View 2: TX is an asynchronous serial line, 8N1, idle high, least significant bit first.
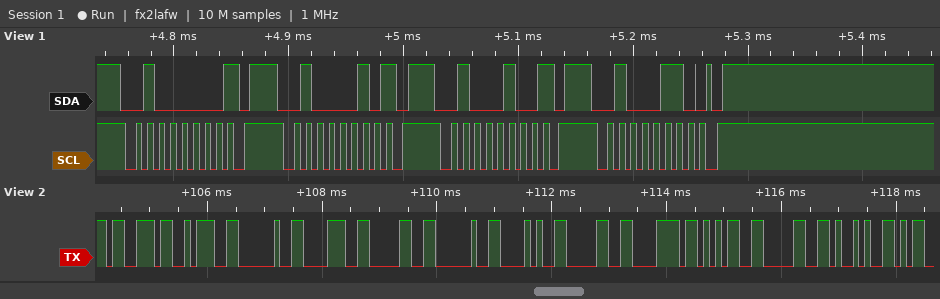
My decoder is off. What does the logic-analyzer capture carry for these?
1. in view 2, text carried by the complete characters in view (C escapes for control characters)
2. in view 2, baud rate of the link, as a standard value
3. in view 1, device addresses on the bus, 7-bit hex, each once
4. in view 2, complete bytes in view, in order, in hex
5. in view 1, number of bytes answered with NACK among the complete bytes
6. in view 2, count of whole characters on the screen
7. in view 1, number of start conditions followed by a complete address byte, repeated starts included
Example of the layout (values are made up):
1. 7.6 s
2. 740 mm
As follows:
1. "s: 80 (0x50)"
2. 9600 baud
3. 0x20 0x21 0x22 0x23
4. 73 3A 20 38 30 20 28 30 78 35 30 29
5. 3
6. 12
7. 4
